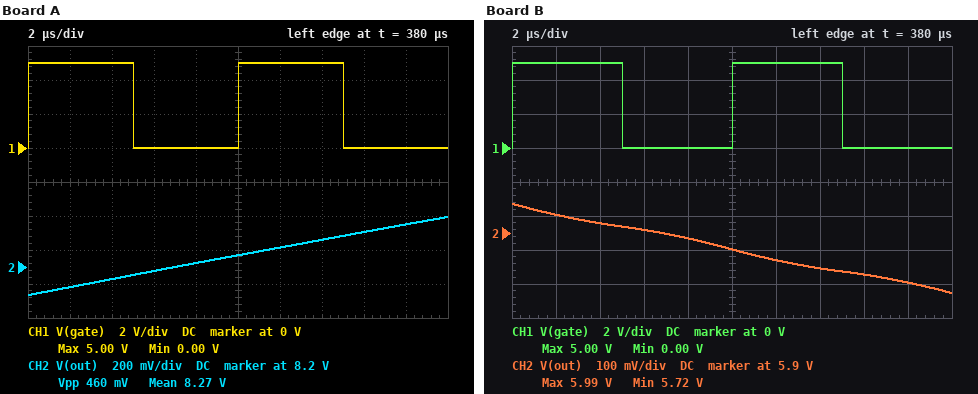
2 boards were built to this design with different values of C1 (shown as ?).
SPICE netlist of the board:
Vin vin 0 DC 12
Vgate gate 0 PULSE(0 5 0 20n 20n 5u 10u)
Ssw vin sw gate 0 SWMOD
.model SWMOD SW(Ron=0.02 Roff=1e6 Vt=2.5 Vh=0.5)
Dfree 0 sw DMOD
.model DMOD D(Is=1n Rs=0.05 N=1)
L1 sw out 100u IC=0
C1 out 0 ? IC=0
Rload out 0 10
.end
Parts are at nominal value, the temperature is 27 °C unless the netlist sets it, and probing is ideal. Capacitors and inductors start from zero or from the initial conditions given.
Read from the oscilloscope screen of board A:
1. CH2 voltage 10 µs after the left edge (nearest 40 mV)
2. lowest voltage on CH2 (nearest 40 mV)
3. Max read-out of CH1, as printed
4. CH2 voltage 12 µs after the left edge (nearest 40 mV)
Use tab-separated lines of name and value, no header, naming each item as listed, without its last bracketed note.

CH2 voltage 10 µs after the left edge	8.28 V
lowest voltage on CH2	8.04 V
Max read-out of CH1, as printed	5.00 V
CH2 voltage 12 µs after the left edge	8.32 V
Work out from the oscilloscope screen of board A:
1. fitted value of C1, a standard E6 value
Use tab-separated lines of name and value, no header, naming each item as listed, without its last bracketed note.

fitted value of C1, a standard E6 value	330 µF
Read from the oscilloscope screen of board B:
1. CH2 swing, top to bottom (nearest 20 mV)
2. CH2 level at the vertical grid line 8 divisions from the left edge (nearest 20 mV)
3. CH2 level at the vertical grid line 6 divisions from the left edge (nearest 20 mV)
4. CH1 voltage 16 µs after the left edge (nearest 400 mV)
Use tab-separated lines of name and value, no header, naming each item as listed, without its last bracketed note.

CH2 swing, top to bottom	260 mV
CH2 level at the vertical grid line 8 divisions from the left edge	5.78 V
CH2 level at the vertical grid line 6 divisions from the left edge	5.82 V
CH1 voltage 16 µs after the left edge	0 V
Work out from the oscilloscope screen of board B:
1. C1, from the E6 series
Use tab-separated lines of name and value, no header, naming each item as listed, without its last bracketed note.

C1, from the E6 series	33 µF
